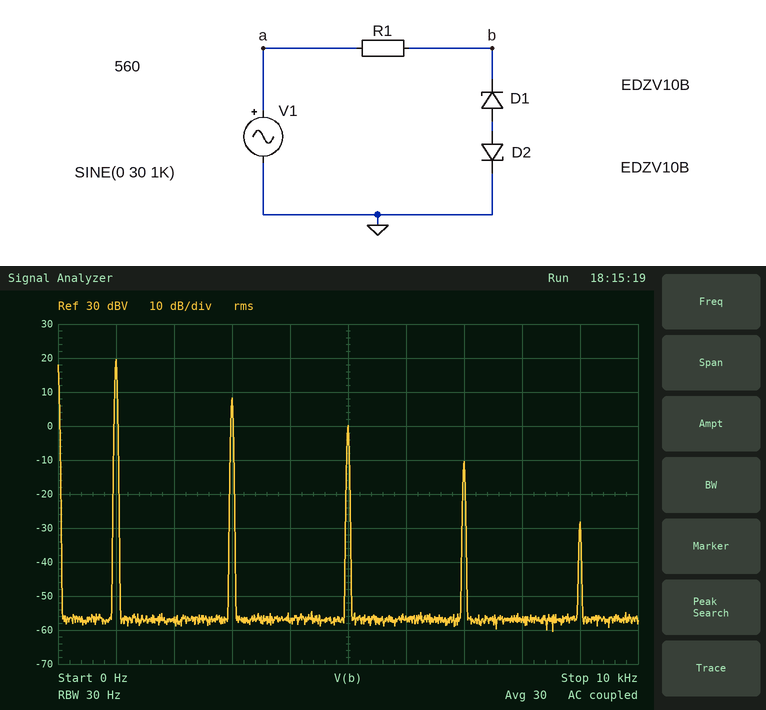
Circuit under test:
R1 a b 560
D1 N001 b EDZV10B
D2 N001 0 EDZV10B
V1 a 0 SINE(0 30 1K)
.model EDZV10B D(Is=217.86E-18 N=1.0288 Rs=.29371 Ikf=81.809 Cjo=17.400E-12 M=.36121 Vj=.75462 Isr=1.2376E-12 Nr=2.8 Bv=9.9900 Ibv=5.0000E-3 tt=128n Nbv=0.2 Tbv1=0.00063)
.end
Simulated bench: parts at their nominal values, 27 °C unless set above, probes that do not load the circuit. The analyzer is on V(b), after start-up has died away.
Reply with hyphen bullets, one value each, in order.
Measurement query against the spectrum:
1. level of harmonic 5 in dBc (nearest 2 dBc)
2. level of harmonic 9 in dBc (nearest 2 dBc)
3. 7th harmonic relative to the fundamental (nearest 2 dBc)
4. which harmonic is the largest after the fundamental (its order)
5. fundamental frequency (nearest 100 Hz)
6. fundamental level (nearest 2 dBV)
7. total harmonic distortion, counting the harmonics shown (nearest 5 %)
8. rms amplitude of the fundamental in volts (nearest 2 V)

- -20 dBc
- -48 dBc
- -30 dBc
- 3
- 1.0 kHz
- 20 dBV
- 30 %
- 10 V
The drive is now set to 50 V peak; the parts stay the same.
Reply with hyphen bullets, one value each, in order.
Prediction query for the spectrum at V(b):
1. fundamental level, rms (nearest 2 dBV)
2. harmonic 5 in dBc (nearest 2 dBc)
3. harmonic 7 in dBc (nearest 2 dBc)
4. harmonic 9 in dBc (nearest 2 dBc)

- 20 dBV
- -16 dBc
- -20 dBc
- -26 dBc
